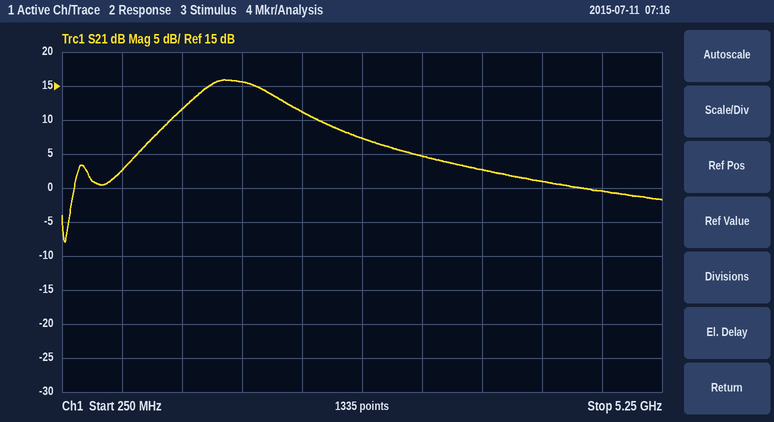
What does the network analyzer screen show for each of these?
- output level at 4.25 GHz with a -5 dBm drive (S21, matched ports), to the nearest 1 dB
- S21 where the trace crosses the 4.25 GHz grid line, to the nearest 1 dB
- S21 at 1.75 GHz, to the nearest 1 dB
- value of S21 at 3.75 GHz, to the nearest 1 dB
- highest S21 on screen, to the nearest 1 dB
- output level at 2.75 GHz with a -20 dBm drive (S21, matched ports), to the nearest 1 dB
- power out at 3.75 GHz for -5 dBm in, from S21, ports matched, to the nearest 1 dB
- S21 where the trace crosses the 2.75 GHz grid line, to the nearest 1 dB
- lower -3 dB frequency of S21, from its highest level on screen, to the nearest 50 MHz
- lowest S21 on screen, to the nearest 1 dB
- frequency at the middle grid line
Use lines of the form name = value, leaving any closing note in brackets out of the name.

output level at 4.25 GHz with a -5 dBm drive (S21, matched ports), to the nearest 1 dB = -4 dBm
S21 where the trace crosses the 4.25 GHz grid line, to the nearest 1 dB = 1 dB
S21 at 1.75 GHz, to the nearest 1 dB = 16 dB
value of S21 at 3.75 GHz, to the nearest 1 dB = 3 dB
highest S21 on screen, to the nearest 1 dB = 16 dB
output level at 2.75 GHz with a -20 dBm drive (S21, matched ports), to the nearest 1 dB = -13 dBm
power out at 3.75 GHz for -5 dBm in, from S21, ports matched, to the nearest 1 dB = -2 dBm
S21 where the trace crosses the 2.75 GHz grid line, to the nearest 1 dB = 7 dB
lower -3 dB frequency of S21, from its highest level on screen, to the nearest 50 MHz = 1.35 GHz
lowest S21 on screen, to the nearest 1 dB = -8 dB
frequency at the middle grid line = 2.75 GHz
